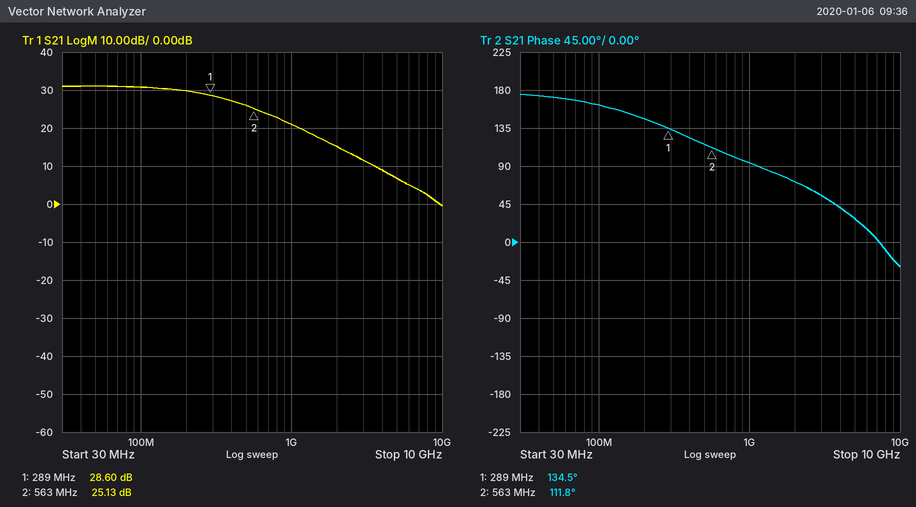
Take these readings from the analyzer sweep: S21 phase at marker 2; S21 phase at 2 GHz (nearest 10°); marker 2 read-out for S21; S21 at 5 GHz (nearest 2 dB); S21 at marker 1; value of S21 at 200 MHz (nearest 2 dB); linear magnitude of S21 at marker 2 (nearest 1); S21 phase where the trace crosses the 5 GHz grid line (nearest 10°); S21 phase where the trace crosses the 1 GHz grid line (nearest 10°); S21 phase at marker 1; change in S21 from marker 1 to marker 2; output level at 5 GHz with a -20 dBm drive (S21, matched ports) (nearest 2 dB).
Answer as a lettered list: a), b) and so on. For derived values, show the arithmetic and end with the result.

a) 111.8°
b) 70°
c) 25.13 dB
d) 6 dB
e) 28.60 dB
f) 30 dB
g) 10^(25.13/20) ≈ 18
h) 30°
i) 90°
j) 134.5°
k) 25.13 − (28.6) = -3.47 dB
l) -20 dBm + (6 dB) = -14 dBm
